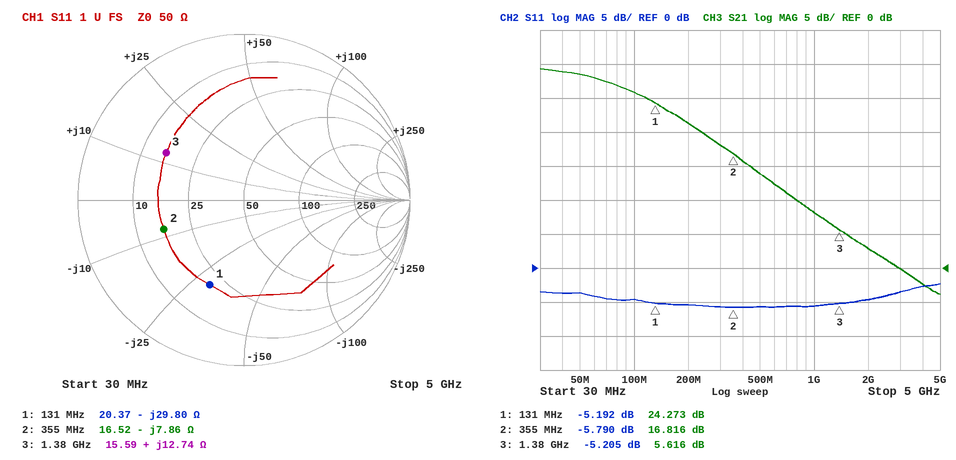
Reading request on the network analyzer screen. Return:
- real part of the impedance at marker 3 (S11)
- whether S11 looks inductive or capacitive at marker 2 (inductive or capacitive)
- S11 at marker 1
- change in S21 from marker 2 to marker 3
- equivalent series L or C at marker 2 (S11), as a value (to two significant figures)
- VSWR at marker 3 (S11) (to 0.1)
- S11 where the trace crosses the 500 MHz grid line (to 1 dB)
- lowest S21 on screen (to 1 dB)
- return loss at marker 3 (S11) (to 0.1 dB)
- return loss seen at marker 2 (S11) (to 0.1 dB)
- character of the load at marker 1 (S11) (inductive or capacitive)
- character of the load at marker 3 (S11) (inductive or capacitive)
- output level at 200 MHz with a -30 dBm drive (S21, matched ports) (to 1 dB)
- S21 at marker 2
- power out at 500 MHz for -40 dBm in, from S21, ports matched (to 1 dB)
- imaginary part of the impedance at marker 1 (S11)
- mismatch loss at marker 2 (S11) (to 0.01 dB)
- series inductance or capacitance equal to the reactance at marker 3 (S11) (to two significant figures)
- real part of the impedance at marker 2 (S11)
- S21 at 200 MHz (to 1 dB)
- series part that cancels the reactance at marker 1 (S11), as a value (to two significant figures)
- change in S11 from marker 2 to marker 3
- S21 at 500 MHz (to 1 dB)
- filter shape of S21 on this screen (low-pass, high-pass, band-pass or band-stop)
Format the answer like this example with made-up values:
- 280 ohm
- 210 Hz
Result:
- 15.59 Ω
- capacitive
- -5.192 dB
- -11.200 dB
- 57 pF
- 3.4
- -6 dB
- -4 dB
- 5.2 dB
- 5.8 dB
- capacitive
- inductive
- -9 dBm
- 16.816 dB
- -26 dBm
- -29.80 Ω
- 1.33 dB
- 1.5 nH
- 16.52 Ω
- 21 dB
- 36 nH
- 0.585 dB
- 14 dB
- low-pass
